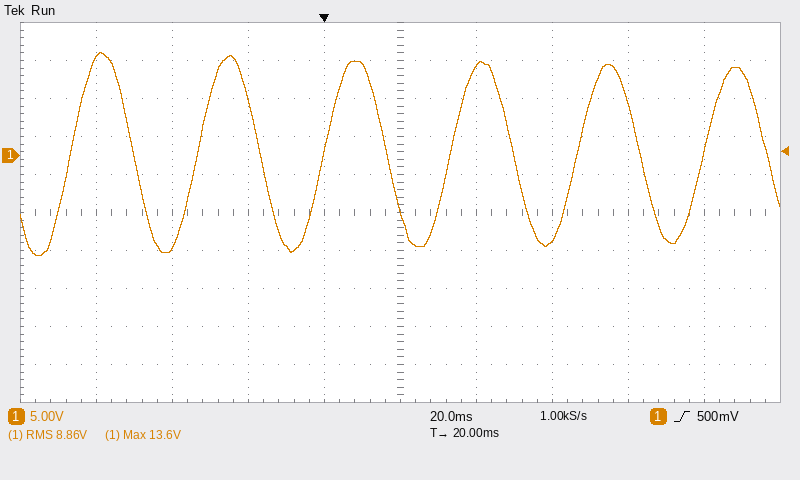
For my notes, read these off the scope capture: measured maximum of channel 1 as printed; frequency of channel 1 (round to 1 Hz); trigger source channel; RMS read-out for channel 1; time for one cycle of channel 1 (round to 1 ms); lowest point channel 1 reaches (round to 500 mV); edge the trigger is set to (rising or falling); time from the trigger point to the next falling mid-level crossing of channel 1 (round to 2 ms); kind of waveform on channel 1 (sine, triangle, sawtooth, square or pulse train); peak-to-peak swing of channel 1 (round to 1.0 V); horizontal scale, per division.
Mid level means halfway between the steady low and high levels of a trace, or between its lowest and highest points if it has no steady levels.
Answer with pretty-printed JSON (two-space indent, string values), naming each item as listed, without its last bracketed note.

{
  "measured maximum of channel 1 as printed": "13.6 V",
  "frequency of channel 1": "30 Hz",
  "trigger source channel": "channel 1",
  "RMS read-out for channel 1": "8.86 V",
  "time for one cycle of channel 1": "33 ms",
  "lowest point channel 1 reaches": "-13.0 V",
  "edge the trigger is set to": "rising",
  "time from the trigger point to the next falling mid-level crossing of channel 1": "16 ms",
  "kind of waveform on channel 1": "sine",
  "peak-to-peak swing of channel 1": "27.0 V",
  "horizontal scale, per division": "20 ms"
}
